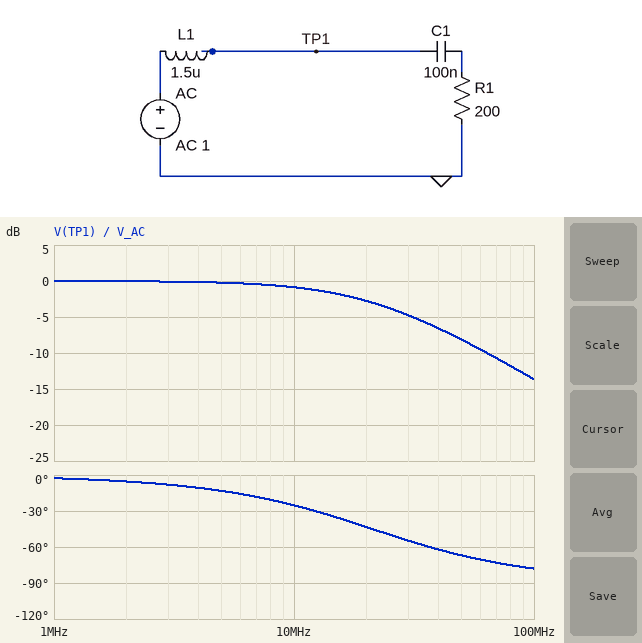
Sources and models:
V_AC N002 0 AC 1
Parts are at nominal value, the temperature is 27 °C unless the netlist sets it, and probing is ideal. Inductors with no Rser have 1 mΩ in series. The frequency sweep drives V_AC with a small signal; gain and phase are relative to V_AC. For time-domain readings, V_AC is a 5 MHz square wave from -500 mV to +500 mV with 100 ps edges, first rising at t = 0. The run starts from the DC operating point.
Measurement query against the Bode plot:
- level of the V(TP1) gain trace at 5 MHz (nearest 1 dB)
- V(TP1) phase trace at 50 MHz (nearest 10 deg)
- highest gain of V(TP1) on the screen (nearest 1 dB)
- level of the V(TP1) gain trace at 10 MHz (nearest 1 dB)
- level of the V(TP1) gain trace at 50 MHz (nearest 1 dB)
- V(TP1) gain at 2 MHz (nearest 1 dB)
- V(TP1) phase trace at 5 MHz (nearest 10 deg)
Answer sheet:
0 dB
-70 deg
0 dB
-1 dB
-8 dB
0 dB
-10 deg
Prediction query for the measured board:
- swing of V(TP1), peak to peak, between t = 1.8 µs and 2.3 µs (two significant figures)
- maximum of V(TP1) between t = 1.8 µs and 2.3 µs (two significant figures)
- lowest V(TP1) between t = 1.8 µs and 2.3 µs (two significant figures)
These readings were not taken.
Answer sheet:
1.0 V
500 mV
-500 mV
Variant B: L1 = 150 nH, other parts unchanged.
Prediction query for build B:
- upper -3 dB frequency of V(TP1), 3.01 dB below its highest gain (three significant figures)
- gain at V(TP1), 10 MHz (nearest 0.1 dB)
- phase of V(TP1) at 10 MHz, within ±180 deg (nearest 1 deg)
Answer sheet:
212 MHz
0 dB
-3 deg
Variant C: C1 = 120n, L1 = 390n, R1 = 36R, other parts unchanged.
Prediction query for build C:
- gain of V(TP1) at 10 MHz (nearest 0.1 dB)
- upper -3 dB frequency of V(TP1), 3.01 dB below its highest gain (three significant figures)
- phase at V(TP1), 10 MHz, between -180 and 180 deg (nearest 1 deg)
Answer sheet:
-1.6 dB
14.7 MHz
-34 deg
